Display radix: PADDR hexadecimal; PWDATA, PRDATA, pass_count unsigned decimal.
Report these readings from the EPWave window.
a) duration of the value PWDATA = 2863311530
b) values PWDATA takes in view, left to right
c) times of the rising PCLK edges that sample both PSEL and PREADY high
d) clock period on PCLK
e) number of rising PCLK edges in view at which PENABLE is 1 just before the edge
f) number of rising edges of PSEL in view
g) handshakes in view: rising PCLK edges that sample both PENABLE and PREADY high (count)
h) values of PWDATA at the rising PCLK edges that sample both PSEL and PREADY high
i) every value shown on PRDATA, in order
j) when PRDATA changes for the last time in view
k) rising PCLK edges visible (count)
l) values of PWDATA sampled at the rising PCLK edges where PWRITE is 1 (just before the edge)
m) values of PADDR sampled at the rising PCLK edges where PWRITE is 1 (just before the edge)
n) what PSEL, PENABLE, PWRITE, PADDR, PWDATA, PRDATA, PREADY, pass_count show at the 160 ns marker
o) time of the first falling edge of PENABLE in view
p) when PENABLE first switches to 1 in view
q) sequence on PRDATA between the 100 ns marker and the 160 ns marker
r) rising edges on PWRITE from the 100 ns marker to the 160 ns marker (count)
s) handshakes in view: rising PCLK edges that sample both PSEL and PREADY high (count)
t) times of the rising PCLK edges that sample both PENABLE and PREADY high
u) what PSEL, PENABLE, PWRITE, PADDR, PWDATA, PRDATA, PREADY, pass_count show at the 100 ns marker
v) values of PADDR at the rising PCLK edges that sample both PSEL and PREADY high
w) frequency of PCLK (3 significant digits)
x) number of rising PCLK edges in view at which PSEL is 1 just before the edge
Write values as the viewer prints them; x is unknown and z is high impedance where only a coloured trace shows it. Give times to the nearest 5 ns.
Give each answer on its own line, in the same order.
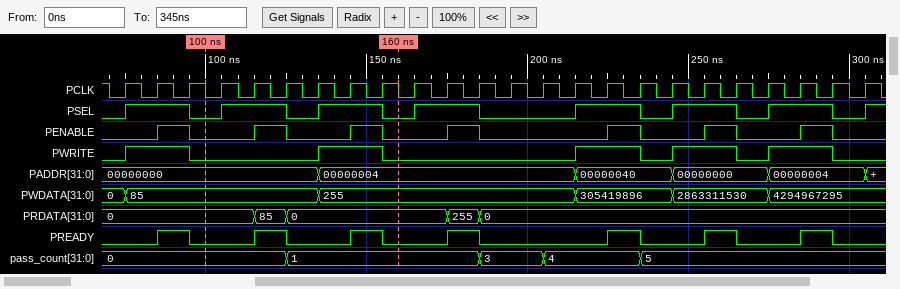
30 ns
0, 85, 255, 305419896, 2863311530, 4294967295
95 ns, 125 ns, 155 ns, 185 ns, 235 ns, 265 ns, 295 ns
10 ns
7
8
7
85, 85, 255, 255, 305419896, 2863311530, 4294967295
0, 85, 0, 255, 0
185 ns
24
85, 85, 255, 255, 305419896, 305419896, 2863311530, 2863311530, 4294967295, 4294967295
00000000, 00000000, 00000004, 00000004, 00000040, 00000040, 00000000, 00000000, 00000004, 00000004
PSEL=0, PENABLE=0, PWRITE=0, PADDR=00000004, PWDATA=255, PRDATA=0, PREADY=0, pass_count=1
95 ns
85 ns
0, 85, 0
1
7
95 ns, 125 ns, 155 ns, 185 ns, 235 ns, 265 ns, 295 ns
PSEL=0, PENABLE=0, PWRITE=0, PADDR=00000000, PWDATA=85, PRDATA=0, PREADY=0, pass_count=0
00000000, 00000000, 00000004, 00000004, 00000040, 00000000, 00000004
100 MHz
14
